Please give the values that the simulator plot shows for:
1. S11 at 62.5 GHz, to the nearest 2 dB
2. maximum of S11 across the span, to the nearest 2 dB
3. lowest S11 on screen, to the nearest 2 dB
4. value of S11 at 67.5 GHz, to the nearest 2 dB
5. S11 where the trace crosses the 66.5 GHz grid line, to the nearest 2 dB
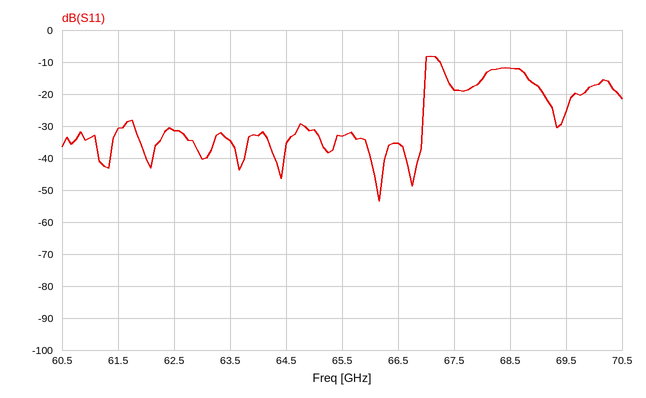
-32 dB
-8 dB
-54 dB
-18 dB
-36 dB
